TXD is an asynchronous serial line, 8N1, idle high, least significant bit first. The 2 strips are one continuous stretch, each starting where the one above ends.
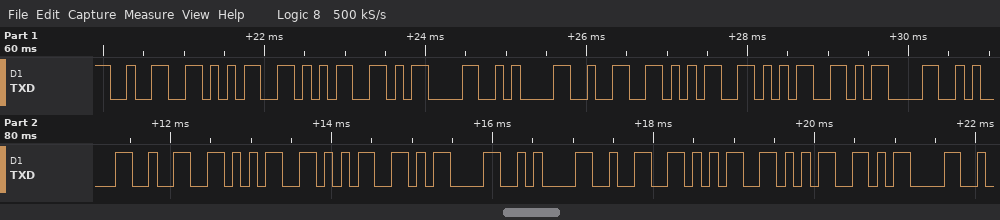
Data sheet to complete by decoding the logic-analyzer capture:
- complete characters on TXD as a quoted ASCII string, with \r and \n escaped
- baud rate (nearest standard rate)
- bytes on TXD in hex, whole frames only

"255\r\n255\r\n255\r\n255\r"
9600 baud
32 35 35 0D 0A 32 35 35 0D 0A 32 35 35 0D 0A 32 35 35 0D
